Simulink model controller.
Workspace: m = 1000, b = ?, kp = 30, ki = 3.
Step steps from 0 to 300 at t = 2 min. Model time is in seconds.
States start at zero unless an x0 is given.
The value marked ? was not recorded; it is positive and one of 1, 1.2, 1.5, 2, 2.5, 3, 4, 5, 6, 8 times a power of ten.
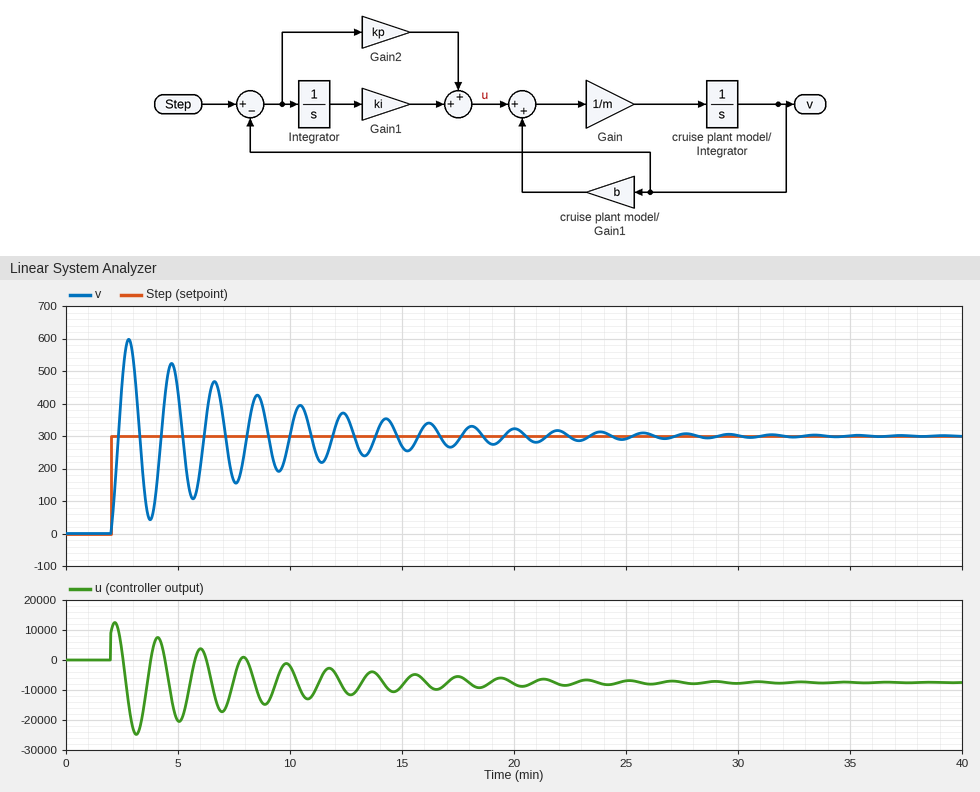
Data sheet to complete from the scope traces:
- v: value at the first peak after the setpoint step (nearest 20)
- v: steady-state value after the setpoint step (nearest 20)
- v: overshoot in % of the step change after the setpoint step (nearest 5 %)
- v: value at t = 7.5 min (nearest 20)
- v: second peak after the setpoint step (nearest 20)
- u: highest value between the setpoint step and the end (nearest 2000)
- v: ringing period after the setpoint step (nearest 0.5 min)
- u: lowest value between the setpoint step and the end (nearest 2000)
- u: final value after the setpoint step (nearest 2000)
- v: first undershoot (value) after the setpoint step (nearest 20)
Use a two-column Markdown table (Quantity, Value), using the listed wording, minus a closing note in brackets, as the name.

| Quantity | Value |
|---|---|
| v: value at the first peak after the setpoint step | 600 |
| v: steady-state value after the setpoint step | 300 |
| v: overshoot in % of the step change after the setpoint step | 100 % |
| v: value at t = 7.5 min | 160 |
| v: second peak after the setpoint step | 520 |
| u: highest value between the setpoint step and the end | 12000 |
| v: ringing period after the setpoint step | 2.0 min |
| u: lowest value between the setpoint step and the end | -24000 |
| u: final value after the setpoint step | -8000 |
| v: first undershoot (value) after the setpoint step | 40 |
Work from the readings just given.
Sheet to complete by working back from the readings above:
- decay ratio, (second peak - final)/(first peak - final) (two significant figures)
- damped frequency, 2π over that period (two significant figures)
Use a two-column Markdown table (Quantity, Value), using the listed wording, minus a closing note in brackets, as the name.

| Quantity | Value |
|---|---|
| decay ratio, (second peak - final)/(first peak - final) | 0.73 |
| damped frequency, 2π over that period | 3.1 rad/min |
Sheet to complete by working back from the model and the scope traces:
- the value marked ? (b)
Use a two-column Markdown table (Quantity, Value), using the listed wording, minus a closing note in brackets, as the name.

| Quantity | Value |
|---|---|
| the value marked ? | 25 |
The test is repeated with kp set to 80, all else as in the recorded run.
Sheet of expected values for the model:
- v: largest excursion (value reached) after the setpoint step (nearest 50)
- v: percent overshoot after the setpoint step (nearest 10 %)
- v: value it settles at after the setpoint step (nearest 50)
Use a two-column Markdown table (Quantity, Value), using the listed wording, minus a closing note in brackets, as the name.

| Quantity | Value |
|---|---|
| v: largest excursion (value reached) after the setpoint step | 450 |
| v: percent overshoot after the setpoint step | 50 % |
| v: value it settles at after the setpoint step | 300 |
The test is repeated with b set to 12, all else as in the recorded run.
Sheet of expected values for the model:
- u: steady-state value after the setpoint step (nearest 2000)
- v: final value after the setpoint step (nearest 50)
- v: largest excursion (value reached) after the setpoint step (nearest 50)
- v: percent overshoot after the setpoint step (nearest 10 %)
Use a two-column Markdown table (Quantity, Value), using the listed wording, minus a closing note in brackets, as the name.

| Quantity | Value |
|---|---|
| u: steady-state value after the setpoint step | -4000 |
| v: final value after the setpoint step | 300 |
| v: largest excursion (value reached) after the setpoint step | 500 |
| v: percent overshoot after the setpoint step | 70 % |
